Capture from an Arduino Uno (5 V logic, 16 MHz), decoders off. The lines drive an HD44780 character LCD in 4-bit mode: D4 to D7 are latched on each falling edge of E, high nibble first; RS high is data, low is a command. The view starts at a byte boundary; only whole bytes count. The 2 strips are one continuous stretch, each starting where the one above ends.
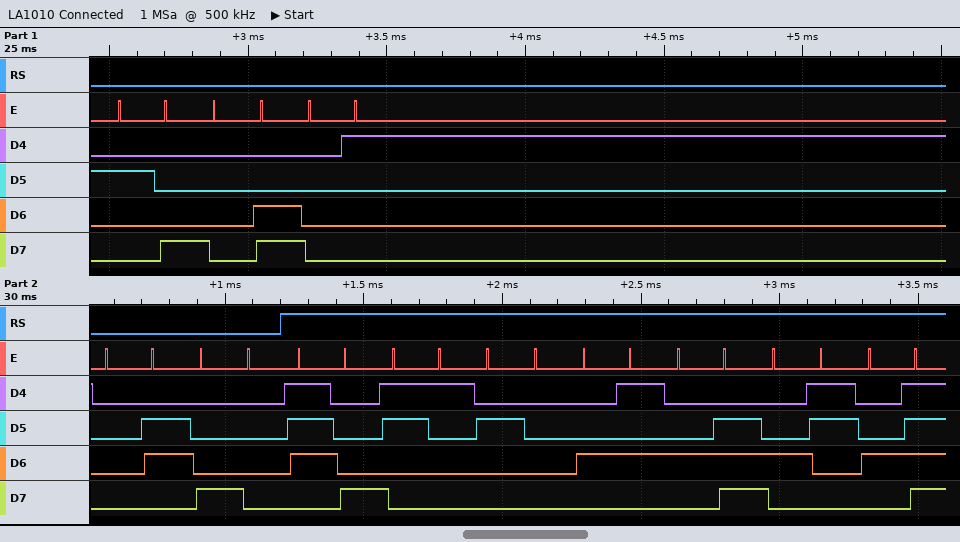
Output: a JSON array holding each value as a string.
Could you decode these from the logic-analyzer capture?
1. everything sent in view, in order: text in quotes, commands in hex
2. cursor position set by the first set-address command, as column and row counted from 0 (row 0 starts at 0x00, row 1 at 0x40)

["0x28 0x0C 0x01 0x06 0x80 \"x1 ENCO\"", "column 0, row 0"]
